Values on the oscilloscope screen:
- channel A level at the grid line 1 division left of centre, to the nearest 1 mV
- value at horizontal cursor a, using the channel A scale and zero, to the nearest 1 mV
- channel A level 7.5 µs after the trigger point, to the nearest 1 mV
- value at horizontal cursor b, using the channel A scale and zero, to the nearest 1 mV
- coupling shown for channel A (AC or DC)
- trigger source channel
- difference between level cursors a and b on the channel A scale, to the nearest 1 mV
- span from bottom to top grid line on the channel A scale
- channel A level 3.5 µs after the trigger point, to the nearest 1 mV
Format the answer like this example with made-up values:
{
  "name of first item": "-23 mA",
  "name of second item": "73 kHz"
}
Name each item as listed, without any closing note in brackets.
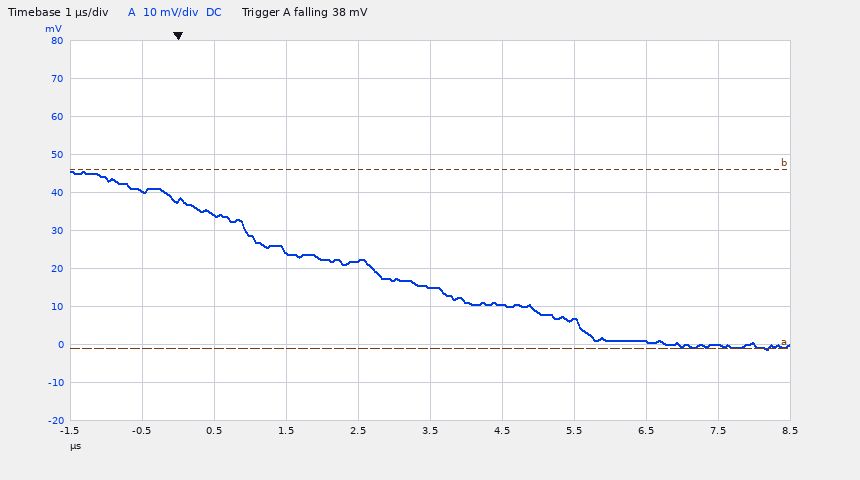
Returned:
{
  "channel A level at the grid line 1 division left of centre, to the nearest 1 mV": "22 mV",
  "value at horizontal cursor a, using the channel A scale and zero, to the nearest 1 mV": "-1 mV",
  "channel A level 7.5 µs after the trigger point, to the nearest 1 mV": "0 mV",
  "value at horizontal cursor b, using the channel A scale and zero, to the nearest 1 mV": "46 mV",
  "coupling shown for channel A": "DC",
  "trigger source channel": "channel A",
  "difference between level cursors a and b on the channel A scale, to the nearest 1 mV": "47 mV",
  "span from bottom to top grid line on the channel A scale": "100 mV",
  "channel A level 3.5 µs after the trigger point, to the nearest 1 mV": "15 mV"
}
